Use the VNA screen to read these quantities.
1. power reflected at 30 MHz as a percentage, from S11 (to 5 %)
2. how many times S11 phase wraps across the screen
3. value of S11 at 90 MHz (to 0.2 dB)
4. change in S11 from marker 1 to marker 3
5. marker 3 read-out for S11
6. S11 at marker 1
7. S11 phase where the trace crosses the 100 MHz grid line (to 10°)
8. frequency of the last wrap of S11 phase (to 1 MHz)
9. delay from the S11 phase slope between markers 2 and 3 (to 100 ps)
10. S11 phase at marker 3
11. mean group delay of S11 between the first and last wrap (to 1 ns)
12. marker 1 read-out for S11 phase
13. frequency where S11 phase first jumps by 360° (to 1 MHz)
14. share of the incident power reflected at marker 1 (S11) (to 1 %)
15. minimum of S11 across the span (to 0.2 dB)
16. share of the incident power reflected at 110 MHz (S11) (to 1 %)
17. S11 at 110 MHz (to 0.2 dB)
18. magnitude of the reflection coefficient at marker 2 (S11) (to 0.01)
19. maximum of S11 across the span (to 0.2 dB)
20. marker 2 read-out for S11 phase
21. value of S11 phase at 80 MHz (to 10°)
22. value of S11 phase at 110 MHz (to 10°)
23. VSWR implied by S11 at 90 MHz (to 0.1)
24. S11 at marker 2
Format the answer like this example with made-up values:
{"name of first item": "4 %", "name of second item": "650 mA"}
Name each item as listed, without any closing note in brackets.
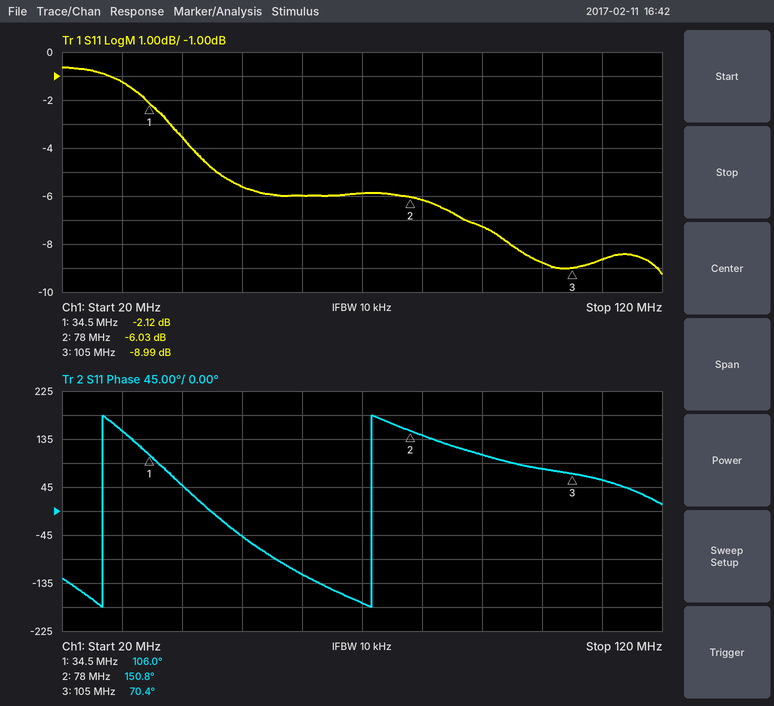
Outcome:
{"power reflected at 30 MHz as a percentage, from S11": "75 %", "how many times S11 phase wraps across the screen": "2", "value of S11 at 90 MHz": "-7.2 dB", "change in S11 from marker 1 to marker 3": "-6.87 dB", "marker 3 read-out for S11": "-8.99 dB", "S11 at marker 1": "-2.12 dB", "S11 phase where the trace crosses the 100 MHz grid line": "80°", "frequency of the last wrap of S11 phase": "72 MHz", "delay from the S11 phase slope between markers 2 and 3": "8.3 ns", "S11 phase at marker 3": "70.4°", "mean group delay of S11 between the first and last wrap": "22 ns", "marker 1 read-out for S11 phase": "106.0°", "frequency where S11 phase first jumps by 360°": "27 MHz", "share of the incident power reflected at marker 1 (S11)": "61 %", "minimum of S11 across the span": "-9.2 dB", "share of the incident power reflected at 110 MHz (S11)": "14 %", "S11 at 110 MHz": "-8.6 dB", "magnitude of the reflection coefficient at marker 2 (S11)": "0.50", "maximum of S11 across the span": "-0.6 dB", "marker 2 read-out for S11 phase": "150.8°", "value of S11 phase at 80 MHz": "140°", "value of S11 phase at 110 MHz": "60°", "VSWR implied by S11 at 90 MHz": "2.5", "S11 at marker 2": "-6.03 dB"}
